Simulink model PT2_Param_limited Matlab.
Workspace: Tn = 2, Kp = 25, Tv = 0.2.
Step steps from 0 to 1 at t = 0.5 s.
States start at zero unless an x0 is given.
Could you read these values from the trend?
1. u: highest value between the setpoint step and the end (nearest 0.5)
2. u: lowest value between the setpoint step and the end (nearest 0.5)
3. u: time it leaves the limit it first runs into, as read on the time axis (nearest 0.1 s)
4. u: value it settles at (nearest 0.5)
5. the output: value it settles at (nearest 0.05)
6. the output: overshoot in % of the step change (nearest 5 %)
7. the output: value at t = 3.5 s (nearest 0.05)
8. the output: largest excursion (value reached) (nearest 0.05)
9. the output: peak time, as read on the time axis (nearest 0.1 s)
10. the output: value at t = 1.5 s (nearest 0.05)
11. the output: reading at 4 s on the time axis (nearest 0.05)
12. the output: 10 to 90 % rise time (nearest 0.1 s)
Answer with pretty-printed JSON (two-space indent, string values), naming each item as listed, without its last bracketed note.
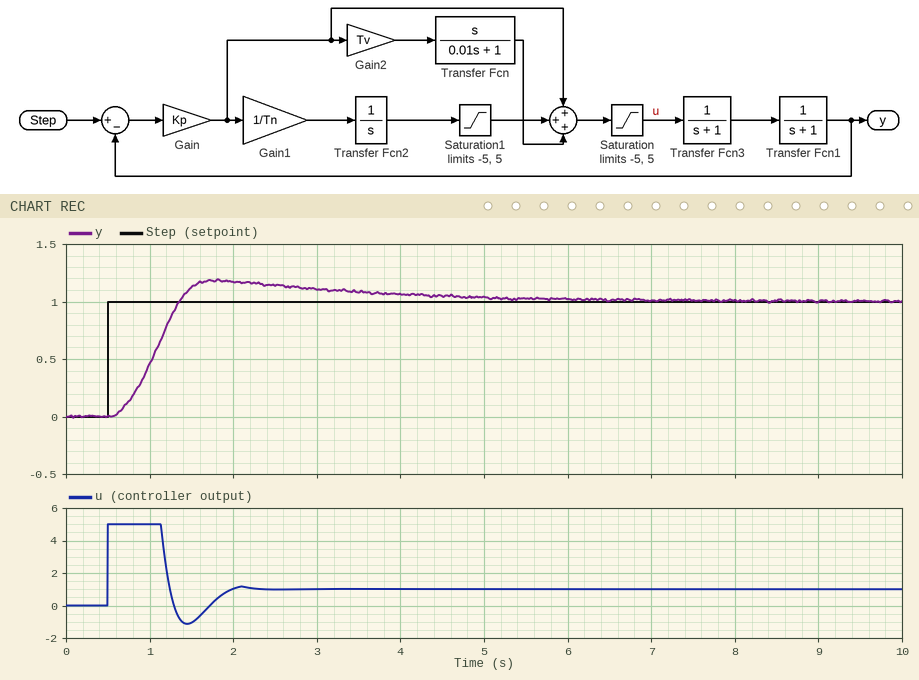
{
  "u: highest value between the setpoint step and the end": "5.0",
  "u: lowest value between the setpoint step and the end": "-1.0",
  "u: time it leaves the limit it first runs into, as read on the time axis": "1.1 s",
  "u: value it settles at": "1.0",
  "the output: value it settles at": "1.00",
  "the output: overshoot in % of the step change": "20 %",
  "the output: value at t = 3.5 s": "1.10",
  "the output: largest excursion (value reached)": "1.20",
  "the output: peak time, as read on the time axis": "1.8 s",
  "the output: value at t = 1.5 s": "1.10",
  "the output: reading at 4 s on the time axis": "1.05",
  "the output: 10 to 90 % rise time": "0.6 s"
}
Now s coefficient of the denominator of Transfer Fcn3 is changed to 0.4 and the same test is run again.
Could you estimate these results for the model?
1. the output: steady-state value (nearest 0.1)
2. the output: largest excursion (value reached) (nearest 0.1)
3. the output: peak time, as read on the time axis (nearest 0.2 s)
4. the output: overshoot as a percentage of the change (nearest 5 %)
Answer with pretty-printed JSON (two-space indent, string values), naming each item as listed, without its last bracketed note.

{
  "the output: steady-state value": "1.0",
  "the output: largest excursion (value reached)": "1.1",
  "the output: peak time, as read on the time axis": "1.6 s",
  "the output: overshoot as a percentage of the change": "10 %"
}
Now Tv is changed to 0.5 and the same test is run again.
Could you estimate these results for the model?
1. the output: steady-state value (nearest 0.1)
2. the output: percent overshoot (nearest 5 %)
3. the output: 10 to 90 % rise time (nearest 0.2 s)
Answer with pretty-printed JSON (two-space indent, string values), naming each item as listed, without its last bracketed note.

{
  "the output: steady-state value": "1.0",
  "the output: percent overshoot": "15 %",
  "the output: 10 to 90 % rise time": "0.8 s"
}
